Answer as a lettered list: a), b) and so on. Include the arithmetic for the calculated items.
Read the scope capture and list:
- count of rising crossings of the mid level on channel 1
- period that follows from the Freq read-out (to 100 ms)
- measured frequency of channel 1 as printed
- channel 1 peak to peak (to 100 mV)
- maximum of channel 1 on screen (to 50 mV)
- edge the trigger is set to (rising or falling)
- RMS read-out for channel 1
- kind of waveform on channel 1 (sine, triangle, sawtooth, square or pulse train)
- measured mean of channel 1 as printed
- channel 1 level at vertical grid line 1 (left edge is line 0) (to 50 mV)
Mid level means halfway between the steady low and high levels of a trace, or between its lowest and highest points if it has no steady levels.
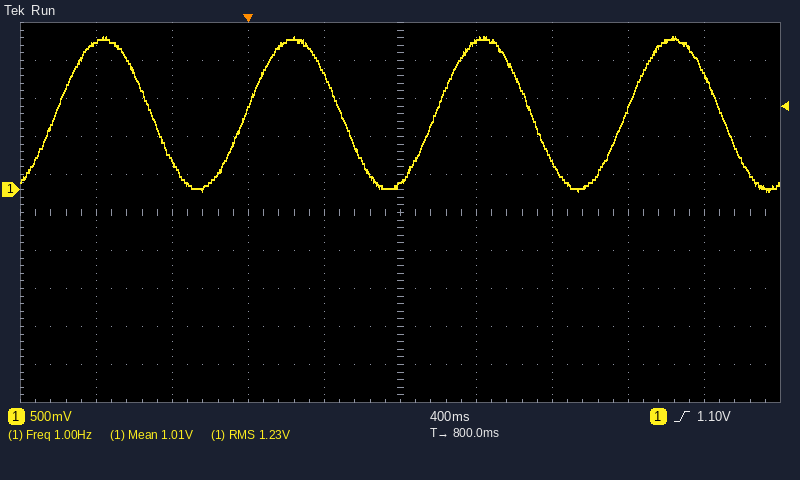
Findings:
a) 4
b) 1 / 1.00 Hz ≈ 1.0 s
c) 1.00 Hz
d) 2.00 V
e) 2.00 V
f) rising
g) 1.23 V
h) sine
i) 1.01 V
j) 1.95 V
